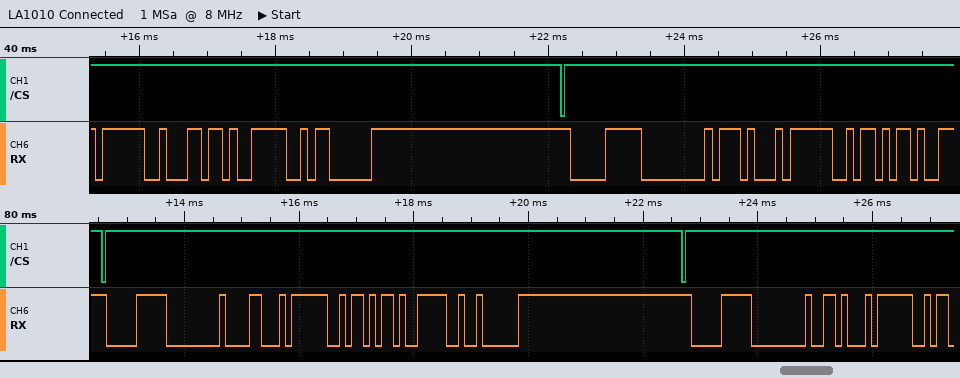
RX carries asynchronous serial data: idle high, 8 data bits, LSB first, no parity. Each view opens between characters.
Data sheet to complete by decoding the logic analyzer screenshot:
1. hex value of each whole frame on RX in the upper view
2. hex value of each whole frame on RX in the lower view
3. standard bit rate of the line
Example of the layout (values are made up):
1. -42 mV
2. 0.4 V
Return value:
1. 3F, 6C, 3E, 03, F0, 00, 17, 3F, 6B
2. F0, 00, 18, 3F, 6B, 3E, 02, F0, 00, 16, 3F
3. 9600 baud
